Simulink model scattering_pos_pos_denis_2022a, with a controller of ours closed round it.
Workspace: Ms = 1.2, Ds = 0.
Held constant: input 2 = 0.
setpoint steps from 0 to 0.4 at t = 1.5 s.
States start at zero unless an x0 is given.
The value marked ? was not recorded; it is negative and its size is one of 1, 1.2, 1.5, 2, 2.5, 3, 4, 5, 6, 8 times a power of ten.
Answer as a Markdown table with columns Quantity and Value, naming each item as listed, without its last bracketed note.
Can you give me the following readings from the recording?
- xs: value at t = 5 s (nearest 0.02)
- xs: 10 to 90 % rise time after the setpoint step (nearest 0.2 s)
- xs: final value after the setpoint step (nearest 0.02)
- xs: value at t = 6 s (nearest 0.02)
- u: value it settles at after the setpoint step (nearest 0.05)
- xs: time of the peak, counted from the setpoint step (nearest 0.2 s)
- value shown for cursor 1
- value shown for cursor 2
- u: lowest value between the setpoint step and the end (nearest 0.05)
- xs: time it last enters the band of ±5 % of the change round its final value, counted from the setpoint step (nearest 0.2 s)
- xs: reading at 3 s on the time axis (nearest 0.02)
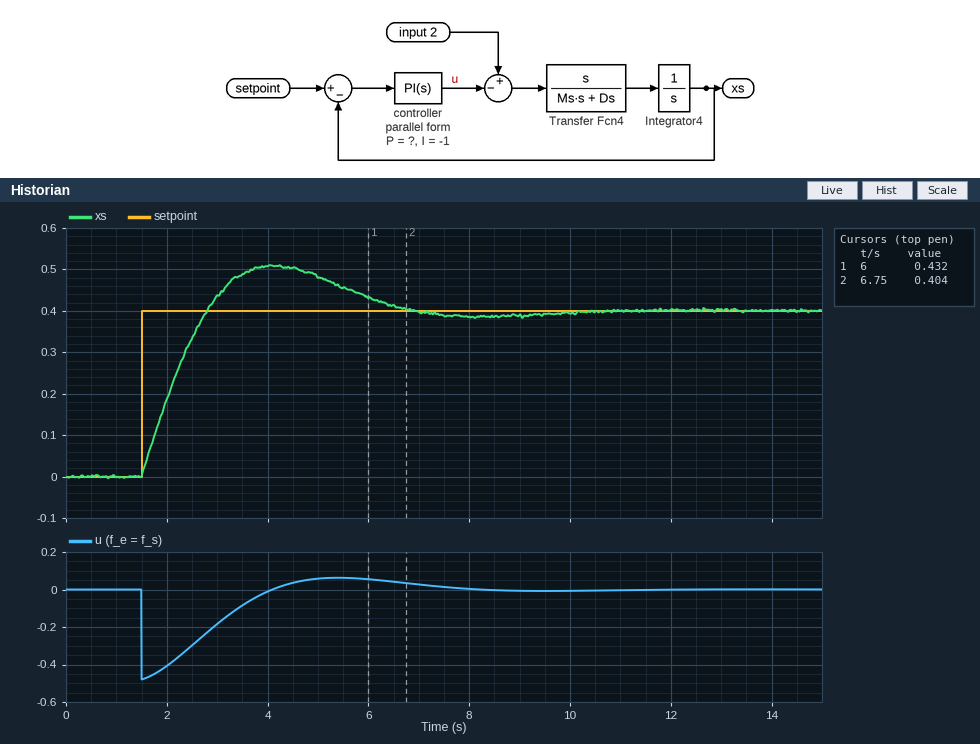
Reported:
| Quantity | Value |
|---|---|
| xs: value at t = 5 s | 0.48 |
| xs: 10 to 90 % rise time after the setpoint step | 1.0 s |
| xs: final value after the setpoint step | 0.40 |
| xs: value at t = 6 s | 0.44 |
| u: value it settles at after the setpoint step | 0.00 |
| xs: time of the peak, counted from the setpoint step | 2.6 s |
| value shown for cursor 1 | 0.432 |
| value shown for cursor 2 | 0.404 |
| u: lowest value between the setpoint step and the end | -0.50 |
| xs: time it last enters the band of ±5 % of the change round its final value, counted from the setpoint step | 4.8 s |
| xs: reading at 3 s on the time axis | 0.44 |
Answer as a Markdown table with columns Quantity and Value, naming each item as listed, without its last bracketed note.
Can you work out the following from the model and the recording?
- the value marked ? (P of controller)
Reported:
| Quantity | Value |
|---|---|
| the value marked ? | -1.2 |
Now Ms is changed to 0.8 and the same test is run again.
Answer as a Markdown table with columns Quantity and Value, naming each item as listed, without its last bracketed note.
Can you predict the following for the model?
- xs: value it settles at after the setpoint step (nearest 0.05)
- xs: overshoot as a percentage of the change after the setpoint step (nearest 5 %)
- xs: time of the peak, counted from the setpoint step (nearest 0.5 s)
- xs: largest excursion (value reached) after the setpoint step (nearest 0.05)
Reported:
| Quantity | Value |
|---|---|
| xs: value it settles at after the setpoint step | 0.40 |
| xs: overshoot as a percentage of the change after the setpoint step | 20 % |
| xs: time of the peak, counted from the setpoint step | 2.0 s |
| xs: largest excursion (value reached) after the setpoint step | 0.50 |
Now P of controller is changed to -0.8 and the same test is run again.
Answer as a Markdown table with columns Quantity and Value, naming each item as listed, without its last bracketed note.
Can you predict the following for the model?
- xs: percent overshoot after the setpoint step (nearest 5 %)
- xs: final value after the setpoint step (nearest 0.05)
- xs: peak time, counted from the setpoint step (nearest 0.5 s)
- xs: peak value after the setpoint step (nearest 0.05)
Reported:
| Quantity | Value |
|---|---|
| xs: percent overshoot after the setpoint step | 40 % |
| xs: final value after the setpoint step | 0.40 |
| xs: peak time, counted from the setpoint step | 3.0 s |
| xs: peak value after the setpoint step | 0.55 |
